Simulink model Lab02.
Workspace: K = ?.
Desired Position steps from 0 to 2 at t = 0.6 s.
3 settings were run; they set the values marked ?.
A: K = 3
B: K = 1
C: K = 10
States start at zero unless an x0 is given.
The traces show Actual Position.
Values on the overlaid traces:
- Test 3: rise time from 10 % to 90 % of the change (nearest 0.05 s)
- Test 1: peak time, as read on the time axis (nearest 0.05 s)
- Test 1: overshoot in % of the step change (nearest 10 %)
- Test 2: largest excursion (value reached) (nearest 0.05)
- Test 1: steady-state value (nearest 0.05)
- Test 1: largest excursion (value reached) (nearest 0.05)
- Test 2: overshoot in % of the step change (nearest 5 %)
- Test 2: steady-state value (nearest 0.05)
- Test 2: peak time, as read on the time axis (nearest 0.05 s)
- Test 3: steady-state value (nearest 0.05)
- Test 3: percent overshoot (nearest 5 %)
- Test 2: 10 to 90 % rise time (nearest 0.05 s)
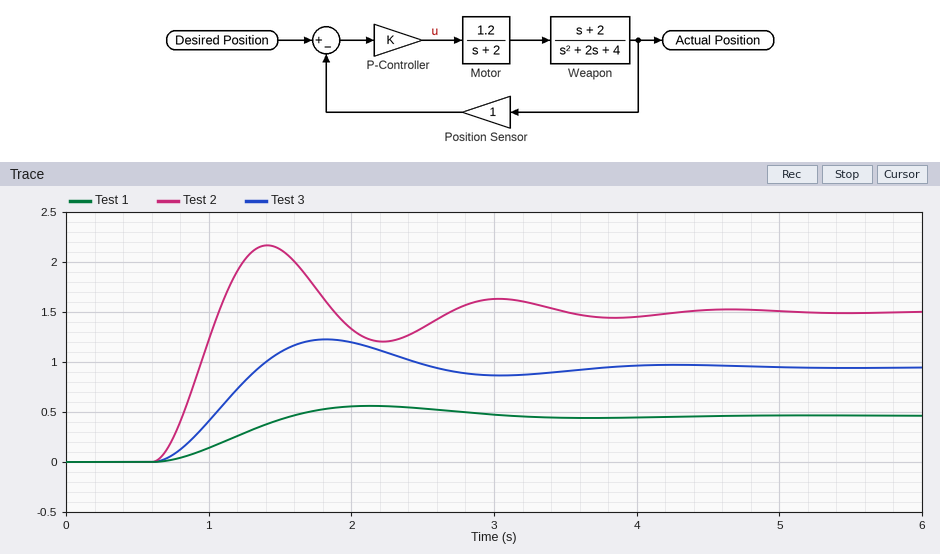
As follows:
0.50 s
2.15 s
20 %
2.15
0.45
0.55
45 %
1.50
1.40 s
0.95
30 %
0.30 s
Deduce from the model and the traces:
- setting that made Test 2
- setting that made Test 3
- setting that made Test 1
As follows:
C
A
B
